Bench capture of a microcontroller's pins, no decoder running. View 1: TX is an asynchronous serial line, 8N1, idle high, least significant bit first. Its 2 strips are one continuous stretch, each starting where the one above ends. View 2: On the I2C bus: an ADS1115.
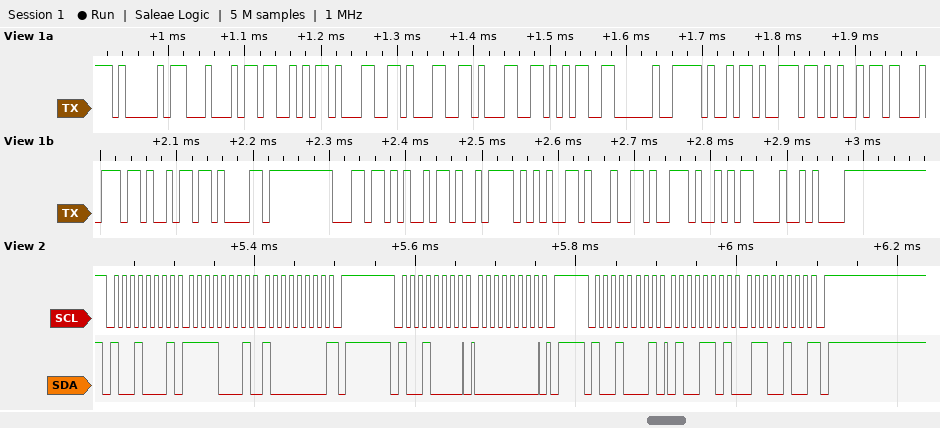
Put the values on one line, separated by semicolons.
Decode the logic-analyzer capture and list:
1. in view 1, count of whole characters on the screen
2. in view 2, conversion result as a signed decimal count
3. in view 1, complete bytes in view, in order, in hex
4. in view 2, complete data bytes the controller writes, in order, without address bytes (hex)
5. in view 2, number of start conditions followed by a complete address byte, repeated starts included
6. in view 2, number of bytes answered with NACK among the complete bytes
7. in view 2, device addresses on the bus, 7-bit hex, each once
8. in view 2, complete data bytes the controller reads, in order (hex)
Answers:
22; 19812; 41 44 53 31 31 31 35 20 69 6E 69 74 69 61 6C 69 7A 65 64 2E 0D 0A; 00; 3; 2; 0x48; F1 80 4D 64
